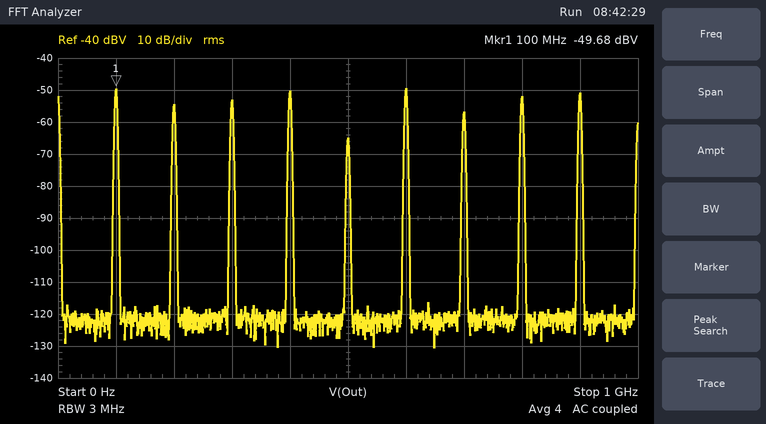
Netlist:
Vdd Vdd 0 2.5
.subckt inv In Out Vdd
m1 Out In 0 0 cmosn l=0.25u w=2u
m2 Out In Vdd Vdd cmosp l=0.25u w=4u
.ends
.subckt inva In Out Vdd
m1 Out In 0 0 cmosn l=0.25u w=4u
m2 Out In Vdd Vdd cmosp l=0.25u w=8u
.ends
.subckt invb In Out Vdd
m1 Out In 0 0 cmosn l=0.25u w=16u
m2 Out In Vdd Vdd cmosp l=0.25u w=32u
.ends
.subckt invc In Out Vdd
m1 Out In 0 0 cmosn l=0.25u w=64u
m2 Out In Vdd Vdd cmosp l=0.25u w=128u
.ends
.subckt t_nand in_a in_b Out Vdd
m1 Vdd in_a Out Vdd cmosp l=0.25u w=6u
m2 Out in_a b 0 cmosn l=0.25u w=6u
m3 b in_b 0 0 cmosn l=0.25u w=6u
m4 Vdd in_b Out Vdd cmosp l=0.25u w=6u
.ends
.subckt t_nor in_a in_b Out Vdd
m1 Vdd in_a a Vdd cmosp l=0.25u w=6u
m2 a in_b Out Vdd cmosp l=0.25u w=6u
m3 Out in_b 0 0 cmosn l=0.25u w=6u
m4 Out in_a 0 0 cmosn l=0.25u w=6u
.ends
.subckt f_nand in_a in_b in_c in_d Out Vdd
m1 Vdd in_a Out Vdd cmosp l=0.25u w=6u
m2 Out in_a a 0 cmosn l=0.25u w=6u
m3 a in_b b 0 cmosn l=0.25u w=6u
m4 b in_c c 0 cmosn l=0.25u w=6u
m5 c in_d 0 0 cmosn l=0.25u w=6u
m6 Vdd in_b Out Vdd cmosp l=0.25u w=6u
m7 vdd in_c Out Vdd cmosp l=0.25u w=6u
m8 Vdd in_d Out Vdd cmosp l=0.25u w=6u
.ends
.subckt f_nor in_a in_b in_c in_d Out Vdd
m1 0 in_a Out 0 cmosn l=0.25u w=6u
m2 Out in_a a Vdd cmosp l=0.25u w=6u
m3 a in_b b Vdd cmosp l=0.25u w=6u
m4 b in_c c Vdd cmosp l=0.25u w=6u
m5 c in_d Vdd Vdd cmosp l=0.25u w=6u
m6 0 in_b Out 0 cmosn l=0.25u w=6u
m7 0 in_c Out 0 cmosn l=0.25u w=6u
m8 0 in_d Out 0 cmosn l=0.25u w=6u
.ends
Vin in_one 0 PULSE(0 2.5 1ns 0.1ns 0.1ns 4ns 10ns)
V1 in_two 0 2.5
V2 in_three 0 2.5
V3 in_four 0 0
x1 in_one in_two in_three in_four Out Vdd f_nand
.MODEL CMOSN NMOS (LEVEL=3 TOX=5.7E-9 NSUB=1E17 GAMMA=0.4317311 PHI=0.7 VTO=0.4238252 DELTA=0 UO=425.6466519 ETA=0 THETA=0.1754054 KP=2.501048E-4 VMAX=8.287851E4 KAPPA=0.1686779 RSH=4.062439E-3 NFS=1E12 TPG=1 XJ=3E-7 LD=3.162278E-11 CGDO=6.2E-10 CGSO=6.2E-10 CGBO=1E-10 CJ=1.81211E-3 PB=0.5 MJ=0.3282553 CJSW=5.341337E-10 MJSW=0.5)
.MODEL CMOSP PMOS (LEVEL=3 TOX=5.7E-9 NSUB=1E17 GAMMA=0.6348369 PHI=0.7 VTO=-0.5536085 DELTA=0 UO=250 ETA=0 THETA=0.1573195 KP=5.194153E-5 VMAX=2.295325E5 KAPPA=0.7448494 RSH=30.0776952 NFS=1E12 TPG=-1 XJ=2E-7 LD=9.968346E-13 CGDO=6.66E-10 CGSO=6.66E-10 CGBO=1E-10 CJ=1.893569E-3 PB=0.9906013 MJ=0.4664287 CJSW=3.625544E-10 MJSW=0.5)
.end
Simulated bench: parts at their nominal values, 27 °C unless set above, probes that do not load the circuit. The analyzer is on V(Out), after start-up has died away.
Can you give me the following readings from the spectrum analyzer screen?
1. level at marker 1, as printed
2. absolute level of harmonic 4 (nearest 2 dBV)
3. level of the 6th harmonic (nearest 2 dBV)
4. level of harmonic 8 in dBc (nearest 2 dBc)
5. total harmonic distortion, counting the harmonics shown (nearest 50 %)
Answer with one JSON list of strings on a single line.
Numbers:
["-49.68 dBV", "-50 dBV", "-50 dBV", "-2 dBc", "200 %"]
